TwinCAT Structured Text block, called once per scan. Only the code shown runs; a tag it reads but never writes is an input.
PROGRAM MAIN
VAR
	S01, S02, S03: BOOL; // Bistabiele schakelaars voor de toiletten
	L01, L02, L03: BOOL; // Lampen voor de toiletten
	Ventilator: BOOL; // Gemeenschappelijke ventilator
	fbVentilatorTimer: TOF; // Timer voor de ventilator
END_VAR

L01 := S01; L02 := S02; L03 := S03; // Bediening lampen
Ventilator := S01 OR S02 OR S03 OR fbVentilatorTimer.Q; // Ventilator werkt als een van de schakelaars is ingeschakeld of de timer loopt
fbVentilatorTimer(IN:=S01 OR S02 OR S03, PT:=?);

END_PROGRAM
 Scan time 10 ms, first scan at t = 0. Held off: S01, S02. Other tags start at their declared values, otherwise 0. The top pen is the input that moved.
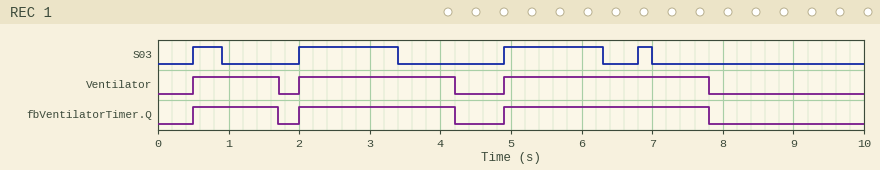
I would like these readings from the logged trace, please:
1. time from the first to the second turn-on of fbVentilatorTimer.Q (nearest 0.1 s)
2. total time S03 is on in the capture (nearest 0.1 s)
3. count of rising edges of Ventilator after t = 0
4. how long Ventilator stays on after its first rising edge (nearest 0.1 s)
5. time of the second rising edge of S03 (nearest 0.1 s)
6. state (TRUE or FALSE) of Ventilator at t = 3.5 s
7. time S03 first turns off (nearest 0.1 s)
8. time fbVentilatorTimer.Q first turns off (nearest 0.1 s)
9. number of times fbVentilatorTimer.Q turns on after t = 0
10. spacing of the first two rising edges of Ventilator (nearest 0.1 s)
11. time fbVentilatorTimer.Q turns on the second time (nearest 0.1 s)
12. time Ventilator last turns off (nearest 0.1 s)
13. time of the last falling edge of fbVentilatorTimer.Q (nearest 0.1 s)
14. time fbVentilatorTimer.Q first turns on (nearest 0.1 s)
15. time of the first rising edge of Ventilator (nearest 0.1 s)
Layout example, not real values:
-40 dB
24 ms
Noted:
1.5 s
3.4 s
3
1.2 s
2.0 s
TRUE
0.9 s
1.7 s
3
1.5 s
2.0 s
7.8 s
7.8 s
0.5 s
0.5 s
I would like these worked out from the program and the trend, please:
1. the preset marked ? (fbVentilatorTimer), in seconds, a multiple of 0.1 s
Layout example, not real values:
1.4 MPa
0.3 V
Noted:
0.8 s
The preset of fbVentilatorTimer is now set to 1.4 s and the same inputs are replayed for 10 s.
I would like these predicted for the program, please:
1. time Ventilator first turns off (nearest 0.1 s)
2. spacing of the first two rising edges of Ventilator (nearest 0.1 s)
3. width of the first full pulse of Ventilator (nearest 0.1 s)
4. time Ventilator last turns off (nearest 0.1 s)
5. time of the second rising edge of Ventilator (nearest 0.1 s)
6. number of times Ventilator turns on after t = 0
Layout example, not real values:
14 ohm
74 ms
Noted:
4.8 s
4.4 s
4.3 s
8.4 s
4.9 s
2
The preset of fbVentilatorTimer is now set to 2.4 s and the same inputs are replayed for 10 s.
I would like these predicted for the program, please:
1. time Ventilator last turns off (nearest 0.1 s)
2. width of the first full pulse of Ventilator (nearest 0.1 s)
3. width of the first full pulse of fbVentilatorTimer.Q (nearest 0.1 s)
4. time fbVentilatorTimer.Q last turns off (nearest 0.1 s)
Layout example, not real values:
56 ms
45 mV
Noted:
9.4 s
8.9 s
8.9 s
9.4 s
